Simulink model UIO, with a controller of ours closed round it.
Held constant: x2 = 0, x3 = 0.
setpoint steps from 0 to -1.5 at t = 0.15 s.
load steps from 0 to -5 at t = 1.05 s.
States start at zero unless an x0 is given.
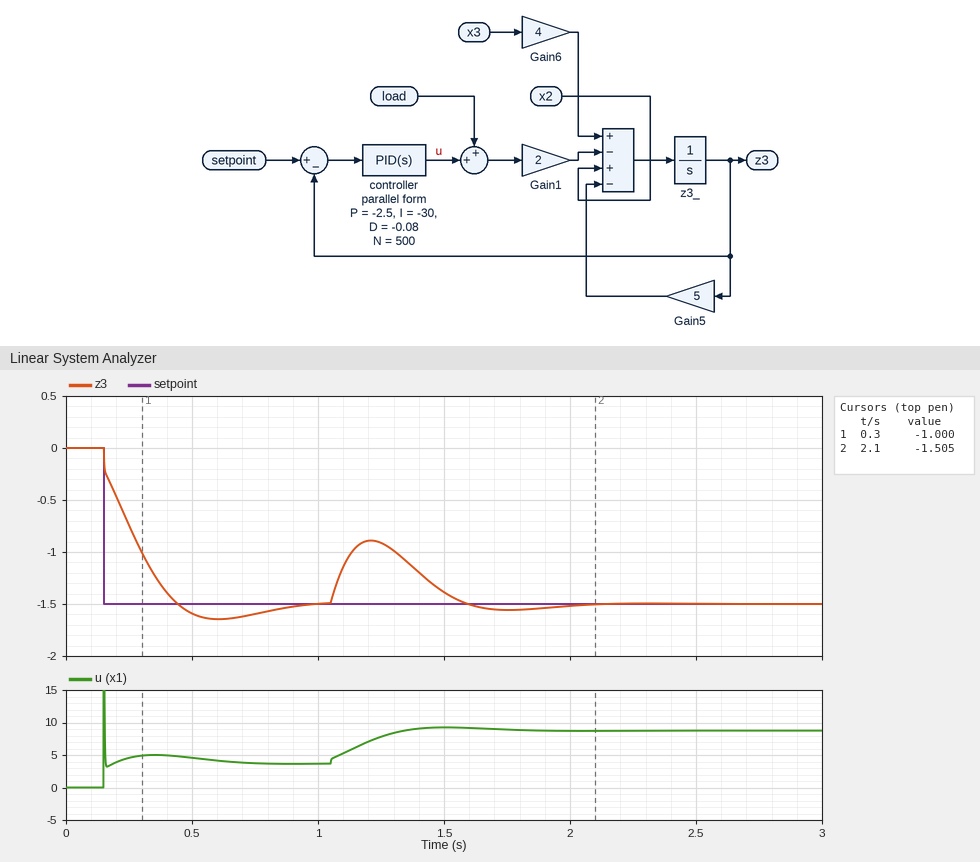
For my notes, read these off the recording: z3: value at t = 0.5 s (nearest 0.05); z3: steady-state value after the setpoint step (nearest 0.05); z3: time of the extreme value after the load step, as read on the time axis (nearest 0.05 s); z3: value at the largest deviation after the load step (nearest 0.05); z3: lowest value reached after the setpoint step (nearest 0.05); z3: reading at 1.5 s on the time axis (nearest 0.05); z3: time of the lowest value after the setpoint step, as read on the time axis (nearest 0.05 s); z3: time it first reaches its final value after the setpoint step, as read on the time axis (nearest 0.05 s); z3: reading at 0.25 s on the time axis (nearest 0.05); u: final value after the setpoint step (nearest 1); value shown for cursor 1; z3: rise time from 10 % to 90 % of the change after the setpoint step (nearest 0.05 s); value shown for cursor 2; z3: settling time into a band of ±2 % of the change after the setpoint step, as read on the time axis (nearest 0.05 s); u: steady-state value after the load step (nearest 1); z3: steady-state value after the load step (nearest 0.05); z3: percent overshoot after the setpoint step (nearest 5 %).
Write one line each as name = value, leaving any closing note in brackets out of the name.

z3: value at t = 0.5 s = -1.60
z3: steady-state value after the setpoint step = -1.50
z3: time of the extreme value after the load step, as read on the time axis = 1.20 s
z3: value at the largest deviation after the load step = -0.90
z3: lowest value reached after the setpoint step = -1.65
z3: reading at 1.5 s on the time axis = -1.40
z3: time of the lowest value after the setpoint step, as read on the time axis = 0.60 s
z3: time it first reaches its final value after the setpoint step, as read on the time axis = 0.45 s
z3: reading at 0.25 s on the time axis = -0.75
u: final value after the setpoint step = 4
value shown for cursor 1 = -1.000
z3: rise time from 10 % to 90 % of the change after the setpoint step = 0.25 s
value shown for cursor 2 = -1.505
z3: settling time into a band of ±2 % of the change after the setpoint step, as read on the time axis = 0.90 s
u: steady-state value after the load step = 9
z3: steady-state value after the load step = -1.50
z3: percent overshoot after the setpoint step = 10 %
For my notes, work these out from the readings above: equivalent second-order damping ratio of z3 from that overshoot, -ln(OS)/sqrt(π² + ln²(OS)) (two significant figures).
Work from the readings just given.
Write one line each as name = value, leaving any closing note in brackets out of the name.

equivalent second-order damping ratio of z3 from that overshoot, -ln(OS)/sqrt(π² + ln²(OS)) = 0.59
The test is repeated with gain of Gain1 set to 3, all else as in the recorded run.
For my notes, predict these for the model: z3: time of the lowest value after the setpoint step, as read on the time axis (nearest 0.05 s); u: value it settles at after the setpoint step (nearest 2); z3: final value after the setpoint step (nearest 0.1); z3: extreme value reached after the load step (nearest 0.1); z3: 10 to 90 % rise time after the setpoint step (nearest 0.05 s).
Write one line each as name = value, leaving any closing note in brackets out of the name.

z3: time of the lowest value after the setpoint step, as read on the time axis = 0.50 s
u: value it settles at after the setpoint step = 2
z3: final value after the setpoint step = -1.5
z3: extreme value reached after the load step = -0.8
z3: 10 to 90 % rise time after the setpoint step = 0.20 s
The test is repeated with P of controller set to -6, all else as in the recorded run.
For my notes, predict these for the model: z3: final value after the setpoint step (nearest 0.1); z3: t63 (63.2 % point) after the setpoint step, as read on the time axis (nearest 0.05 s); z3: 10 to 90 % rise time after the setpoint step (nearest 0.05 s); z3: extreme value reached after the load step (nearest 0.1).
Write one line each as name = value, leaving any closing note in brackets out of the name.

z3: final value after the setpoint step = -1.5
z3: t63 (63.2 % point) after the setpoint step, as read on the time axis = 0.25 s
z3: 10 to 90 % rise time after the setpoint step = 0.20 s
z3: extreme value reached after the load step = -1.1
